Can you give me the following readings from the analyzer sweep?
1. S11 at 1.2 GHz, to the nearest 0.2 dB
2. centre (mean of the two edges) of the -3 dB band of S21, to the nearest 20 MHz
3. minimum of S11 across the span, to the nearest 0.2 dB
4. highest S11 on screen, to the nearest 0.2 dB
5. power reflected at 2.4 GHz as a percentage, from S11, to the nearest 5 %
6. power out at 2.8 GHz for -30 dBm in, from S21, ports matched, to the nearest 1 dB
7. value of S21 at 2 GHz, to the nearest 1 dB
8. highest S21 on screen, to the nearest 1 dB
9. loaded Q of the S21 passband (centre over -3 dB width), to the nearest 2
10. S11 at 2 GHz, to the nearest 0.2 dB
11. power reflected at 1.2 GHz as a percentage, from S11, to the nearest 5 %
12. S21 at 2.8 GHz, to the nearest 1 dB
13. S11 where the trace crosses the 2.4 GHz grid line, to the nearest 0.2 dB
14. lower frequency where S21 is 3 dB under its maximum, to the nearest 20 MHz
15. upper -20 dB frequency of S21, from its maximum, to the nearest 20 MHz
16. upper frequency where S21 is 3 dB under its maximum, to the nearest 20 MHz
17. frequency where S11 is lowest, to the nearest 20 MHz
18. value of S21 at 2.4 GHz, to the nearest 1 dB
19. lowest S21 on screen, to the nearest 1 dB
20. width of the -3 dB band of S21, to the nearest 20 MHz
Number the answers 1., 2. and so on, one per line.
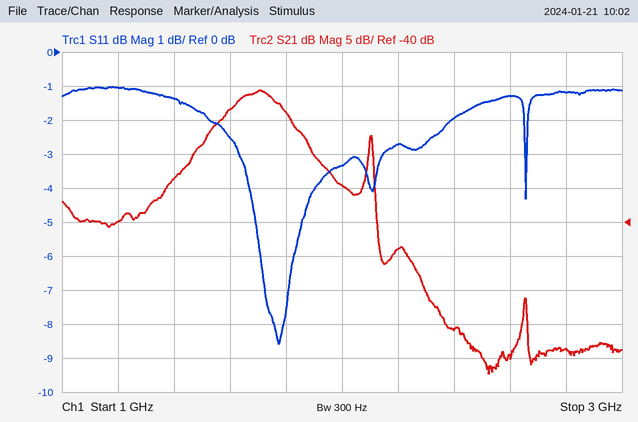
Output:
1. -1.0 dB
2. 1.70 GHz
3. -8.6 dB
4. -1.0 dB
5. 65 %
6. -89 dBm
7. -35 dB
8. -21 dB
9. 8
10. -3.4 dB
11. 80 %
12. -59 dB
13. -2.0 dB
14. 1.60 GHz
15. 2.12 GHz
16. 1.80 GHz
17. 1.78 GHz
18. -56 dB
19. -62 dB
20. 200 MHz
